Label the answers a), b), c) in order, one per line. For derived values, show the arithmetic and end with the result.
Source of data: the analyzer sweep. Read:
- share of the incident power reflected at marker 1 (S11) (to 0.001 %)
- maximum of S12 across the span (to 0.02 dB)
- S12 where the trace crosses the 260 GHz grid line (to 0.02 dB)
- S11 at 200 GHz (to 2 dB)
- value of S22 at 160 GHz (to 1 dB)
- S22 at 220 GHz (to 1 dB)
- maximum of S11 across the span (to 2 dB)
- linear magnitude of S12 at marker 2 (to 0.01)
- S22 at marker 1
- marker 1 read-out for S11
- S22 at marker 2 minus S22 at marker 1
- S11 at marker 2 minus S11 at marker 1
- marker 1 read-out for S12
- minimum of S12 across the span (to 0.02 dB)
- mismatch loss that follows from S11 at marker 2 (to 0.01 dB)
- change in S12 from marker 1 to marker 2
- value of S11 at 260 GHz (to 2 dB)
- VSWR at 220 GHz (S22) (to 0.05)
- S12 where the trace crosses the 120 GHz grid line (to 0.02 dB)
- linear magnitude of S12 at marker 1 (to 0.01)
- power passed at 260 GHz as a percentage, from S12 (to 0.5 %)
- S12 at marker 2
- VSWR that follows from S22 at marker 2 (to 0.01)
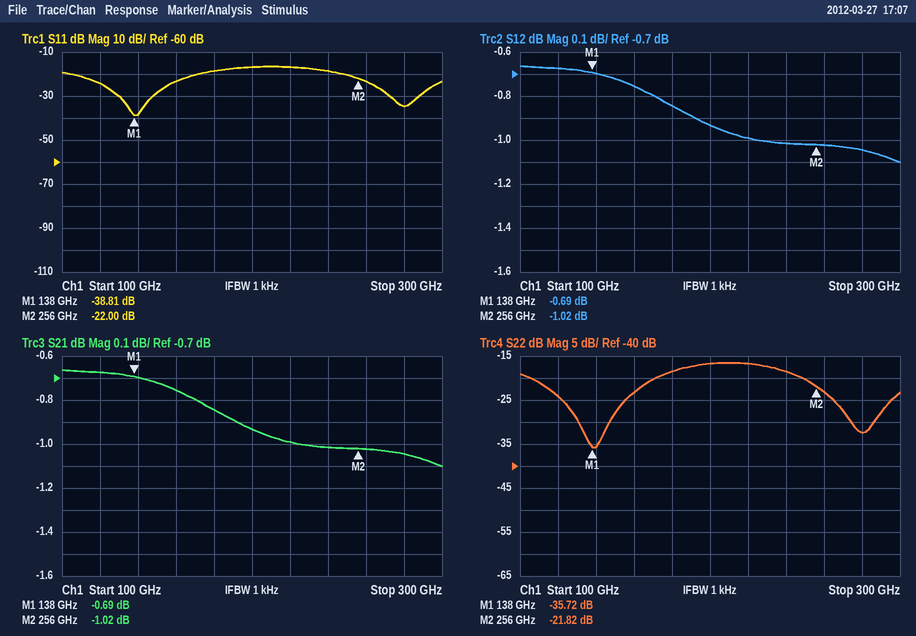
a) 10^(-38.81/10) ≈ 0.013 %
b) -0.66 dB
c) -1.02 dB
d) -16 dB
e) -23 dB
f) -17 dB
g) -16 dB
h) 10^(-1.02/20) ≈ 0.89
i) -35.72 dB
j) -38.81 dB
k) -21.82 − (-35.72) = 13.90 dB
l) -22 − (-38.81) = 16.81 dB
m) -0.69 dB
n) -1.10 dB
o) −10 log10(1 − 10^(-22/10)) ≈ 0.03 dB
p) -1.02 − (-0.69) = -0.33 dB
q) -24 dB
r) |Γ| = 10^(-17/20) = 0.1413; VSWR = (1 + 0.1413)/(1 − 0.1413) ≈ 1.33, so 1.35 to the nearest 0.05
s) -0.68 dB
t) 10^(-0.69/20) ≈ 0.92
u) 10^(-1.02/10) ≈ 79.1 %, so 79.0 % to the nearest 0.5 %
v) -1.02 dB
w) (1 + 0.0811)/(1 − 0.0811) ≈ 1.18
